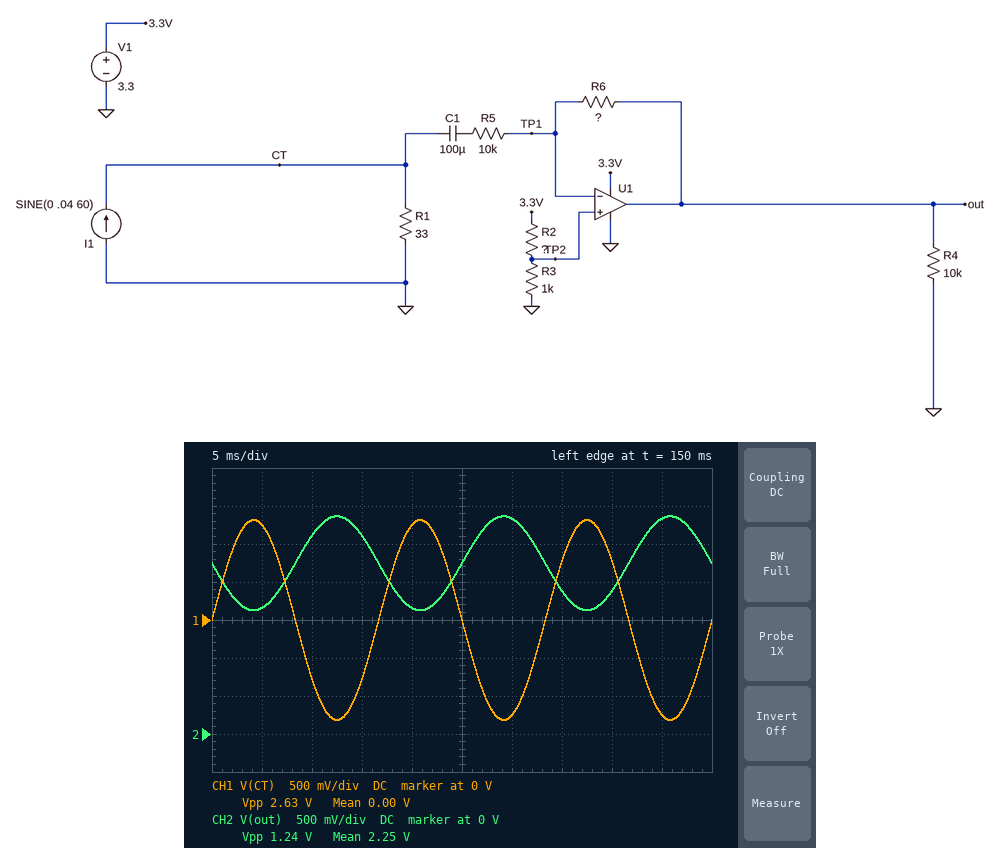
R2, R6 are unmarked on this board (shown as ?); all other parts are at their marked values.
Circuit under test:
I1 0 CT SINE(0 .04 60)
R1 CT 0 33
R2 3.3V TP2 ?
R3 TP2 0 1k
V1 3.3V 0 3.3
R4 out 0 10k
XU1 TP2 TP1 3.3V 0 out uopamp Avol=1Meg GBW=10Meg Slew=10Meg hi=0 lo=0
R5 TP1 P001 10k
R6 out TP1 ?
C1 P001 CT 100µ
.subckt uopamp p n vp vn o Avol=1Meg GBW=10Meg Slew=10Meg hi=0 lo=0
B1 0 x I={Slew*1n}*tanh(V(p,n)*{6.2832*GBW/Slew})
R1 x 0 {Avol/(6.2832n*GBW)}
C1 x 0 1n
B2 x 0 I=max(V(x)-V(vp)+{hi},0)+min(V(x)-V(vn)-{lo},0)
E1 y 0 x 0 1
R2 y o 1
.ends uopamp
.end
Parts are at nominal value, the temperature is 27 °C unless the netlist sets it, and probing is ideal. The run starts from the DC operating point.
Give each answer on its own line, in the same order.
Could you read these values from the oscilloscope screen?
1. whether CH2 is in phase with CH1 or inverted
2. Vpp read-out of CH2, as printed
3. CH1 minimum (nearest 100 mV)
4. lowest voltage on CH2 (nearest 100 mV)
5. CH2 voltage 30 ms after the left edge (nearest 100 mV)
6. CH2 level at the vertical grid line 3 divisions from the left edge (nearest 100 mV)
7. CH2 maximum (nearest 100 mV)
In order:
inverted
1.24 V
-1.3 V
1.6 V
2.8 V
2.6 V
2.9 V
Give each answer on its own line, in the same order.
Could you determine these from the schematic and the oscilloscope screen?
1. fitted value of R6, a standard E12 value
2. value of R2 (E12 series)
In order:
4.7 kΩ
470 Ω
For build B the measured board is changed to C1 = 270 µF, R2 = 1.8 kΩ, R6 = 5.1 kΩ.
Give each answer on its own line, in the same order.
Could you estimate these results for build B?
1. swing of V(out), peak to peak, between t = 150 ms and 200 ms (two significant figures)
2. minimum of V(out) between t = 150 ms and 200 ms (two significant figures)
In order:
1.3 V
510 mV
